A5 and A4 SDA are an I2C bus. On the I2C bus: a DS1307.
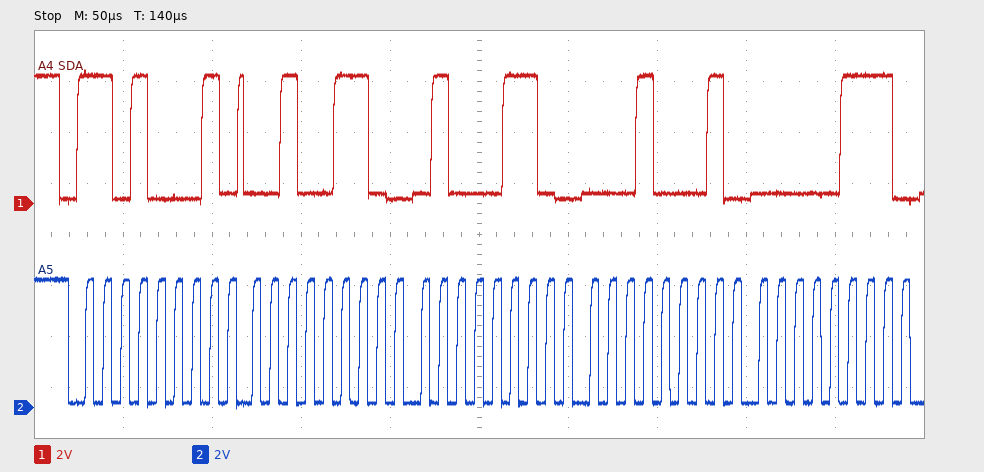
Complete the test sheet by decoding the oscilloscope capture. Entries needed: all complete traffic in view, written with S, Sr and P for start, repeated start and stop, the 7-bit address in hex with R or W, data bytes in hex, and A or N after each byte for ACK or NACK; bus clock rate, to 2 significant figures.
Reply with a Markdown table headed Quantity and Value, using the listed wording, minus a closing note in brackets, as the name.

| Quantity | Value |
|---|---|
| all complete traffic in view, written with S, Sr and P for start, repeated start and stop, the 7-bit address in hex with R or W, data bytes in hex, and A or N after each byte for ACK or NACK | S 68R A 26 A 46 A 11 A 07 A |
| bus clock rate, to 2 significant figures | 100 kHz |
